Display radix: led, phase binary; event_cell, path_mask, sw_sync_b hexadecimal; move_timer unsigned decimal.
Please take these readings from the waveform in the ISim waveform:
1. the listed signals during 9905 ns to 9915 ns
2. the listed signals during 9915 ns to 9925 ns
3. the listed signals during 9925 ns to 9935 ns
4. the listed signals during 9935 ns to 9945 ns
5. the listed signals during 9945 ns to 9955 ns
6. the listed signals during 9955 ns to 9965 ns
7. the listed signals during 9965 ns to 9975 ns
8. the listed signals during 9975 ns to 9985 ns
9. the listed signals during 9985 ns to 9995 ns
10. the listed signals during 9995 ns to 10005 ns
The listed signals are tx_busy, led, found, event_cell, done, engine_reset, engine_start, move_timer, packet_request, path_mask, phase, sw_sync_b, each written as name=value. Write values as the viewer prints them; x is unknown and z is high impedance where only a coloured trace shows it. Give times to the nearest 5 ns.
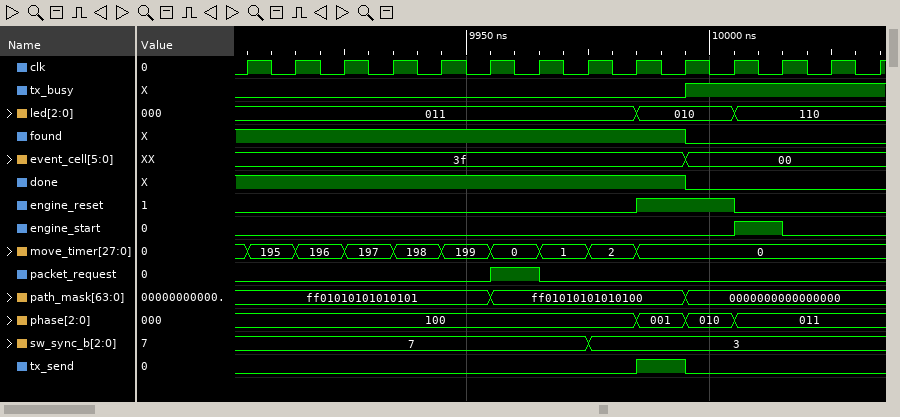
tx_busy=0, led=011, found=1, event_cell=3f, done=1, engine_reset=0, engine_start=0, move_timer=195, packet_request=0, path_mask=ff01010101010101, phase=100, sw_sync_b=7
tx_busy=0, led=011, found=1, event_cell=3f, done=1, engine_reset=0, engine_start=0, move_timer=196, packet_request=0, path_mask=ff01010101010101, phase=100, sw_sync_b=7
tx_busy=0, led=011, found=1, event_cell=3f, done=1, engine_reset=0, engine_start=0, move_timer=197, packet_request=0, path_mask=ff01010101010101, phase=100, sw_sync_b=7
tx_busy=0, led=011, found=1, event_cell=3f, done=1, engine_reset=0, engine_start=0, move_timer=198, packet_request=0, path_mask=ff01010101010101, phase=100, sw_sync_b=7
tx_busy=0, led=011, found=1, event_cell=3f, done=1, engine_reset=0, engine_start=0, move_timer=199, packet_request=0, path_mask=ff01010101010101, phase=100, sw_sync_b=7
tx_busy=0, led=011, found=1, event_cell=3f, done=1, engine_reset=0, engine_start=0, move_timer=0, packet_request=1, path_mask=ff01010101010100, phase=100, sw_sync_b=7
tx_busy=0, led=011, found=1, event_cell=3f, done=1, engine_reset=0, engine_start=0, move_timer=1, packet_request=0, path_mask=ff01010101010100, phase=100, sw_sync_b=7
tx_busy=0, led=011, found=1, event_cell=3f, done=1, engine_reset=0, engine_start=0, move_timer=2, packet_request=0, path_mask=ff01010101010100, phase=100, sw_sync_b=3
tx_busy=0, led=010, found=1, event_cell=3f, done=1, engine_reset=1, engine_start=0, move_timer=0, packet_request=0, path_mask=ff01010101010100, phase=001, sw_sync_b=3
tx_busy=1, led=010, found=0, event_cell=00, done=0, engine_reset=1, engine_start=0, move_timer=0, packet_request=0, path_mask=0000000000000000, phase=010, sw_sync_b=3
